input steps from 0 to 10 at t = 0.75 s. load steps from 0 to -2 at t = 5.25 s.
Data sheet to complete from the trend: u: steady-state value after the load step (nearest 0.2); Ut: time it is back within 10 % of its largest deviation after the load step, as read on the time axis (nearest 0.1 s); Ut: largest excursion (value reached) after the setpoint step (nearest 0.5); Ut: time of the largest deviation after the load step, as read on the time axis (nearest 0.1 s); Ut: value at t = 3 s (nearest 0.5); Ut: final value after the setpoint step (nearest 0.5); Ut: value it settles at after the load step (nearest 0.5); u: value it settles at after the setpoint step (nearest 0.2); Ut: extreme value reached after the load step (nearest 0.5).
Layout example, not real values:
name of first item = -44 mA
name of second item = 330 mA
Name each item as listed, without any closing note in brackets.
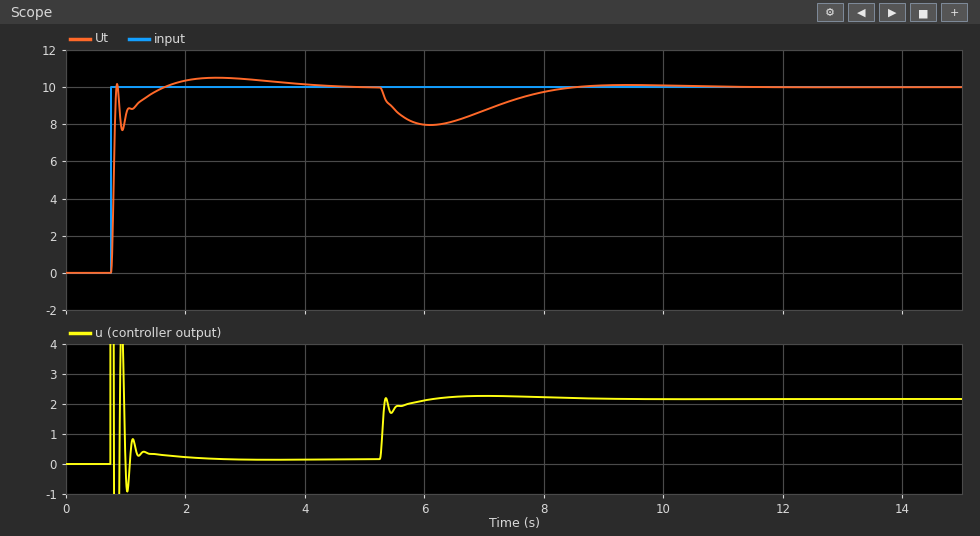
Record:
u: steady-state value after the load step = 2.2
Ut: time it is back within 10 % of its largest deviation after the load step, as read on the time axis = 8.1 s
Ut: largest excursion (value reached) after the setpoint step = 10.5
Ut: time of the largest deviation after the load step, as read on the time axis = 6.1 s
Ut: value at t = 3 s = 10.5
Ut: final value after the setpoint step = 10.0
Ut: value it settles at after the load step = 10.0
u: value it settles at after the setpoint step = 0.2
Ut: extreme value reached after the load step = 8.0
